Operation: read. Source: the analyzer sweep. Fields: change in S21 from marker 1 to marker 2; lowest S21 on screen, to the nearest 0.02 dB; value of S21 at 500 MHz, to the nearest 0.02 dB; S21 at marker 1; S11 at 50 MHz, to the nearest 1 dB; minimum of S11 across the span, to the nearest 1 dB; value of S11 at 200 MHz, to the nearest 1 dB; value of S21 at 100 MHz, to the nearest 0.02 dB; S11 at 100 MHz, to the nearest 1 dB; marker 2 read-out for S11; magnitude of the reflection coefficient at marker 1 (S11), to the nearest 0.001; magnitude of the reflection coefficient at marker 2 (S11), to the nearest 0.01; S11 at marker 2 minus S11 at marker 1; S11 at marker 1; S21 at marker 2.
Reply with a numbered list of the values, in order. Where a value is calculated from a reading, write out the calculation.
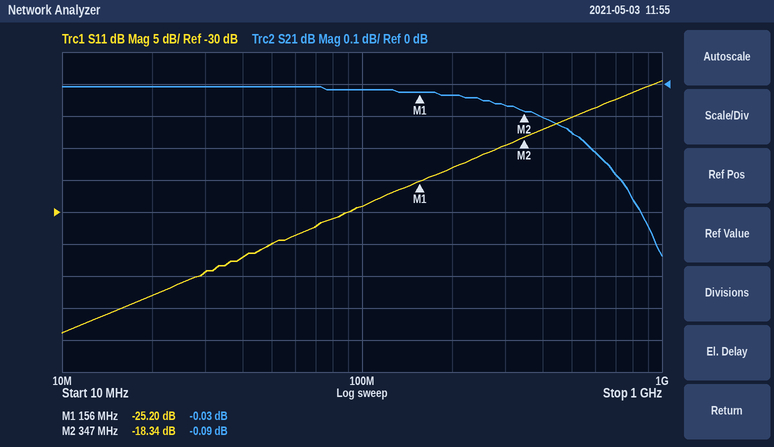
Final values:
1. -0.09 − (-0.03) = -0.06 dB
2. -0.54 dB
3. -0.16 dB
4. -0.03 dB
5. -35 dB
6. -49 dB
7. -23 dB
8. -0.02 dB
9. -29 dB
10. -18.34 dB
11. 10^(-25.2/20) ≈ 0.055
12. 10^(-18.34/20) ≈ 0.12
13. -18.34 − (-25.2) = 6.86 dB
14. -25.20 dB
15. -0.09 dB
